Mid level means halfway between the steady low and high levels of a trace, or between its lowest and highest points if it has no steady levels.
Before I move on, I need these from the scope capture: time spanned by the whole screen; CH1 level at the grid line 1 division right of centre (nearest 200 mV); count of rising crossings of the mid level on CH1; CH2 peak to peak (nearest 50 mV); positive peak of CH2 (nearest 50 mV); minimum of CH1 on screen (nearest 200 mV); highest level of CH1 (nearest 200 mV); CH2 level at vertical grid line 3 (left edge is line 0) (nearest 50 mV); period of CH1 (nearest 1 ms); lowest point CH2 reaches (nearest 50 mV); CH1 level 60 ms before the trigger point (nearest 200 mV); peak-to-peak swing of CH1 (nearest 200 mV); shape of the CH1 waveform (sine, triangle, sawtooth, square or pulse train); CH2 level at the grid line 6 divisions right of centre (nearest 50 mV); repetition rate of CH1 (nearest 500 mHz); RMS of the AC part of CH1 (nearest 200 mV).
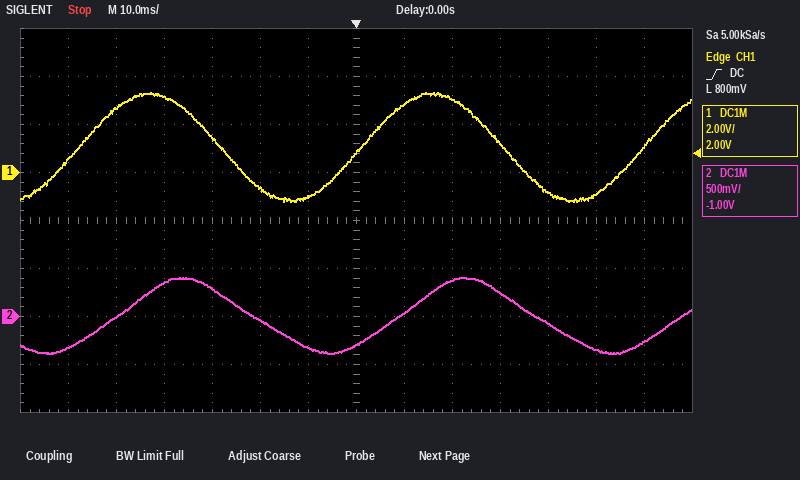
140 ms
2.8 V
3
800 mV
400 mV
-1.2 V
3.4 V
350 mV
59 ms
-400 mV
600 mV
4.6 V
sine
-250 mV
17.0 Hz
1.6 V
